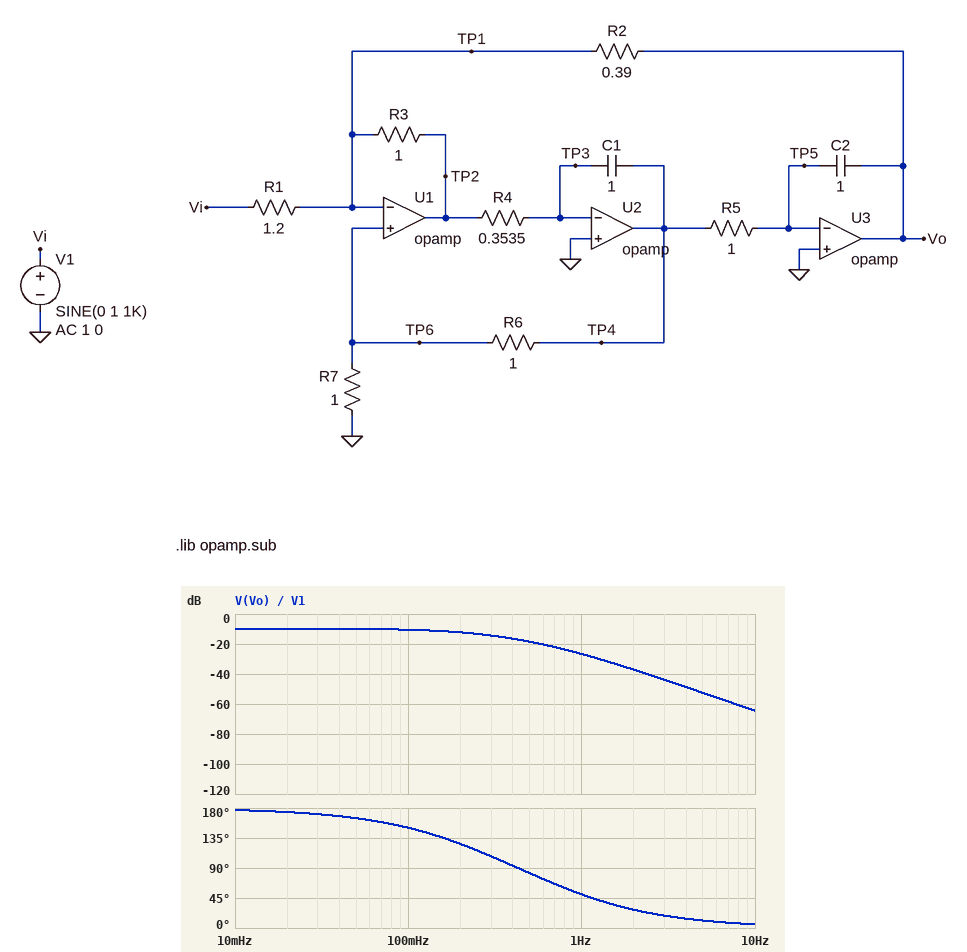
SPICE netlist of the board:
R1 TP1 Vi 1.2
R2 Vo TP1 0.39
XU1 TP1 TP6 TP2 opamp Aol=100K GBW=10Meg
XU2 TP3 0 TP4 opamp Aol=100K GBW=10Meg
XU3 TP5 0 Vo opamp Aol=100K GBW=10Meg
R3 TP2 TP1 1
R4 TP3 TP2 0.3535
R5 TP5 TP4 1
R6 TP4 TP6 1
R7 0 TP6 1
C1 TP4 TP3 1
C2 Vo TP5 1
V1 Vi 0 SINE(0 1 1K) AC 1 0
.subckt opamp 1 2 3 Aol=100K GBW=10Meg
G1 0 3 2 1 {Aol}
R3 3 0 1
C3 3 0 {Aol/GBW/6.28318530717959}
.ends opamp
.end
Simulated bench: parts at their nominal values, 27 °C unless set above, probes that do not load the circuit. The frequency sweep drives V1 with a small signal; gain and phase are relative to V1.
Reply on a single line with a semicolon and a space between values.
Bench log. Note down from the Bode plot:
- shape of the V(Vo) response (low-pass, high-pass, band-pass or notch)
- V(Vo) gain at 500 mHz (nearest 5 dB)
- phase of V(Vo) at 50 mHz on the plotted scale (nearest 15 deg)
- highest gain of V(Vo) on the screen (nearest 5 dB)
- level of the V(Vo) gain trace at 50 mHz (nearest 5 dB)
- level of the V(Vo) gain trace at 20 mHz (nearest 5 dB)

low-pass; -20 dB; 165 deg; -10 dB; -10 dB; -10 dB
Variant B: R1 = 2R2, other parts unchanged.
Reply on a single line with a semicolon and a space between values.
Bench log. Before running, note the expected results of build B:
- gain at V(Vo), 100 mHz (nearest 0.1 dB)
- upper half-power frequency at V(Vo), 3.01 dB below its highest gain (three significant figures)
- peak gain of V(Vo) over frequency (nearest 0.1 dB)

-15.6 dB; 256 mHz; -15.0 dB
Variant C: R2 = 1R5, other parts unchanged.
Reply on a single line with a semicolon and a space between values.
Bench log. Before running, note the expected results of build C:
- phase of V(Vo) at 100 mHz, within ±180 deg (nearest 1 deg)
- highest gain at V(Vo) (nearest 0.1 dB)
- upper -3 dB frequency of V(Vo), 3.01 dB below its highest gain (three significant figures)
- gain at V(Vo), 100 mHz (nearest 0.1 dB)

124 deg; 1.9 dB; 99.4 mHz; -1.1 dB
